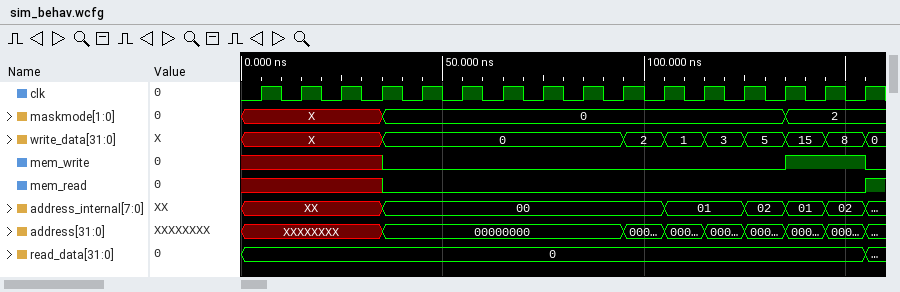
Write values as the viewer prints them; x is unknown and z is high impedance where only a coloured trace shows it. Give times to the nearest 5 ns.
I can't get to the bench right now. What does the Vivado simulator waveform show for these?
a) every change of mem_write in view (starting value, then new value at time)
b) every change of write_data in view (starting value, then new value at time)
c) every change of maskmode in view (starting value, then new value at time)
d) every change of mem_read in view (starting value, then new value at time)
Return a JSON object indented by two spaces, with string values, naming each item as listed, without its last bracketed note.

{
  "every change of mem_write in view": "x, 0 at 35 ns, 1 at 135 ns, 0 at 155 ns",
  "every change of write_data in view": "X, 0 at 35 ns, 2 at 95 ns, 1 at 105 ns, 3 at 115 ns, 5 at 125 ns, 15 at 135 ns, 8 at 145 ns, 0 at 155 ns",
  "every change of maskmode in view": "X, 0 at 35 ns, 2 at 135 ns",
  "every change of mem_read in view": "x, 0 at 35 ns, 1 at 155 ns"
}
